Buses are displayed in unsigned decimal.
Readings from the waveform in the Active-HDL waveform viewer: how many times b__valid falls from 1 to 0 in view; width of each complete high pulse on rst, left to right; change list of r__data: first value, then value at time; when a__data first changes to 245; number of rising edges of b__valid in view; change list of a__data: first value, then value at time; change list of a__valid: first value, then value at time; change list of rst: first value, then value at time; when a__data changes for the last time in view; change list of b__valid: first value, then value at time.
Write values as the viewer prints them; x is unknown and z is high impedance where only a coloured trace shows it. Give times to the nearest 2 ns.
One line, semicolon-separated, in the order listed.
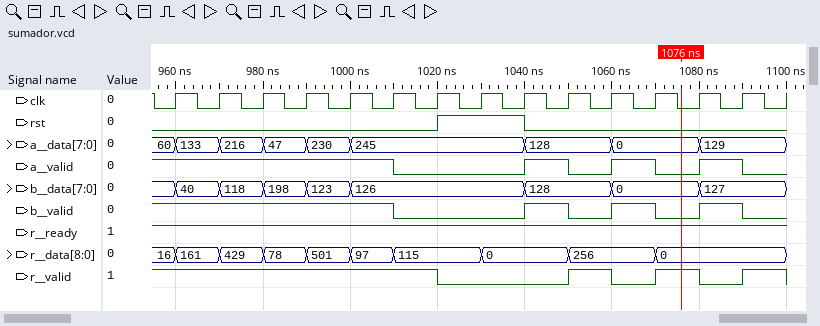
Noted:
4; 20 ns; 16, 161 at 960 ns, 429 at 970 ns, 78 at 980 ns, 501 at 990 ns, 97 at 1000 ns, 115 at 1010 ns, 0 at 1030 ns, 256 at 1050 ns, 0 at 1070 ns; 1000 ns; 3; 60, 133 at 960 ns, 216 at 970 ns, 47 at 980 ns, 230 at 990 ns, 245 at 1000 ns, 128 at 1040 ns, 0 at 1060 ns, 129 at 1080 ns; 1, 0 at 1010 ns, 1 at 1040 ns, 0 at 1050 ns, 1 at 1060 ns, 0 at 1070 ns, 1 at 1080 ns, 0 at 1090 ns; 0, 1 at 1020 ns, 0 at 1040 ns; 1080 ns; 1, 0 at 1010 ns, 1 at 1040 ns, 0 at 1050 ns, 1 at 1060 ns, 0 at 1070 ns, 1 at 1080 ns, 0 at 1090 ns
